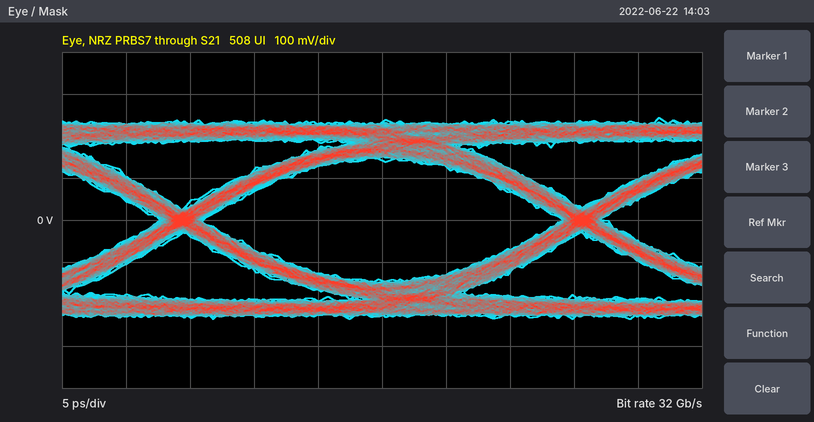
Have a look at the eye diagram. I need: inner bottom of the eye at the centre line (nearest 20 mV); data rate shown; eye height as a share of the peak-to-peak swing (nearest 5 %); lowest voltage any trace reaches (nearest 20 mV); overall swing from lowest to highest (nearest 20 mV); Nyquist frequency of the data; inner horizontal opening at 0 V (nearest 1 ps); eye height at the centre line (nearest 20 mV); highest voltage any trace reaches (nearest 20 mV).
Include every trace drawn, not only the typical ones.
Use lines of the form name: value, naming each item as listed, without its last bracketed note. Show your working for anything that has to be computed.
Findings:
inner bottom of the eye at the centre line: -140 mV
data rate shown: 32 Gb/s
eye height as a share of the peak-to-peak swing: 280 mV / 480 mV ≈ 58.3 %, so 60 % to the nearest 5 %
lowest voltage any trace reaches: -240 mV
overall swing from lowest to highest: 480 mV
Nyquist frequency of the data: 16 GHz
inner horizontal opening at 0 V: 28 ps
eye height at the centre line: 280 mV
highest voltage any trace reaches: 240 mV
